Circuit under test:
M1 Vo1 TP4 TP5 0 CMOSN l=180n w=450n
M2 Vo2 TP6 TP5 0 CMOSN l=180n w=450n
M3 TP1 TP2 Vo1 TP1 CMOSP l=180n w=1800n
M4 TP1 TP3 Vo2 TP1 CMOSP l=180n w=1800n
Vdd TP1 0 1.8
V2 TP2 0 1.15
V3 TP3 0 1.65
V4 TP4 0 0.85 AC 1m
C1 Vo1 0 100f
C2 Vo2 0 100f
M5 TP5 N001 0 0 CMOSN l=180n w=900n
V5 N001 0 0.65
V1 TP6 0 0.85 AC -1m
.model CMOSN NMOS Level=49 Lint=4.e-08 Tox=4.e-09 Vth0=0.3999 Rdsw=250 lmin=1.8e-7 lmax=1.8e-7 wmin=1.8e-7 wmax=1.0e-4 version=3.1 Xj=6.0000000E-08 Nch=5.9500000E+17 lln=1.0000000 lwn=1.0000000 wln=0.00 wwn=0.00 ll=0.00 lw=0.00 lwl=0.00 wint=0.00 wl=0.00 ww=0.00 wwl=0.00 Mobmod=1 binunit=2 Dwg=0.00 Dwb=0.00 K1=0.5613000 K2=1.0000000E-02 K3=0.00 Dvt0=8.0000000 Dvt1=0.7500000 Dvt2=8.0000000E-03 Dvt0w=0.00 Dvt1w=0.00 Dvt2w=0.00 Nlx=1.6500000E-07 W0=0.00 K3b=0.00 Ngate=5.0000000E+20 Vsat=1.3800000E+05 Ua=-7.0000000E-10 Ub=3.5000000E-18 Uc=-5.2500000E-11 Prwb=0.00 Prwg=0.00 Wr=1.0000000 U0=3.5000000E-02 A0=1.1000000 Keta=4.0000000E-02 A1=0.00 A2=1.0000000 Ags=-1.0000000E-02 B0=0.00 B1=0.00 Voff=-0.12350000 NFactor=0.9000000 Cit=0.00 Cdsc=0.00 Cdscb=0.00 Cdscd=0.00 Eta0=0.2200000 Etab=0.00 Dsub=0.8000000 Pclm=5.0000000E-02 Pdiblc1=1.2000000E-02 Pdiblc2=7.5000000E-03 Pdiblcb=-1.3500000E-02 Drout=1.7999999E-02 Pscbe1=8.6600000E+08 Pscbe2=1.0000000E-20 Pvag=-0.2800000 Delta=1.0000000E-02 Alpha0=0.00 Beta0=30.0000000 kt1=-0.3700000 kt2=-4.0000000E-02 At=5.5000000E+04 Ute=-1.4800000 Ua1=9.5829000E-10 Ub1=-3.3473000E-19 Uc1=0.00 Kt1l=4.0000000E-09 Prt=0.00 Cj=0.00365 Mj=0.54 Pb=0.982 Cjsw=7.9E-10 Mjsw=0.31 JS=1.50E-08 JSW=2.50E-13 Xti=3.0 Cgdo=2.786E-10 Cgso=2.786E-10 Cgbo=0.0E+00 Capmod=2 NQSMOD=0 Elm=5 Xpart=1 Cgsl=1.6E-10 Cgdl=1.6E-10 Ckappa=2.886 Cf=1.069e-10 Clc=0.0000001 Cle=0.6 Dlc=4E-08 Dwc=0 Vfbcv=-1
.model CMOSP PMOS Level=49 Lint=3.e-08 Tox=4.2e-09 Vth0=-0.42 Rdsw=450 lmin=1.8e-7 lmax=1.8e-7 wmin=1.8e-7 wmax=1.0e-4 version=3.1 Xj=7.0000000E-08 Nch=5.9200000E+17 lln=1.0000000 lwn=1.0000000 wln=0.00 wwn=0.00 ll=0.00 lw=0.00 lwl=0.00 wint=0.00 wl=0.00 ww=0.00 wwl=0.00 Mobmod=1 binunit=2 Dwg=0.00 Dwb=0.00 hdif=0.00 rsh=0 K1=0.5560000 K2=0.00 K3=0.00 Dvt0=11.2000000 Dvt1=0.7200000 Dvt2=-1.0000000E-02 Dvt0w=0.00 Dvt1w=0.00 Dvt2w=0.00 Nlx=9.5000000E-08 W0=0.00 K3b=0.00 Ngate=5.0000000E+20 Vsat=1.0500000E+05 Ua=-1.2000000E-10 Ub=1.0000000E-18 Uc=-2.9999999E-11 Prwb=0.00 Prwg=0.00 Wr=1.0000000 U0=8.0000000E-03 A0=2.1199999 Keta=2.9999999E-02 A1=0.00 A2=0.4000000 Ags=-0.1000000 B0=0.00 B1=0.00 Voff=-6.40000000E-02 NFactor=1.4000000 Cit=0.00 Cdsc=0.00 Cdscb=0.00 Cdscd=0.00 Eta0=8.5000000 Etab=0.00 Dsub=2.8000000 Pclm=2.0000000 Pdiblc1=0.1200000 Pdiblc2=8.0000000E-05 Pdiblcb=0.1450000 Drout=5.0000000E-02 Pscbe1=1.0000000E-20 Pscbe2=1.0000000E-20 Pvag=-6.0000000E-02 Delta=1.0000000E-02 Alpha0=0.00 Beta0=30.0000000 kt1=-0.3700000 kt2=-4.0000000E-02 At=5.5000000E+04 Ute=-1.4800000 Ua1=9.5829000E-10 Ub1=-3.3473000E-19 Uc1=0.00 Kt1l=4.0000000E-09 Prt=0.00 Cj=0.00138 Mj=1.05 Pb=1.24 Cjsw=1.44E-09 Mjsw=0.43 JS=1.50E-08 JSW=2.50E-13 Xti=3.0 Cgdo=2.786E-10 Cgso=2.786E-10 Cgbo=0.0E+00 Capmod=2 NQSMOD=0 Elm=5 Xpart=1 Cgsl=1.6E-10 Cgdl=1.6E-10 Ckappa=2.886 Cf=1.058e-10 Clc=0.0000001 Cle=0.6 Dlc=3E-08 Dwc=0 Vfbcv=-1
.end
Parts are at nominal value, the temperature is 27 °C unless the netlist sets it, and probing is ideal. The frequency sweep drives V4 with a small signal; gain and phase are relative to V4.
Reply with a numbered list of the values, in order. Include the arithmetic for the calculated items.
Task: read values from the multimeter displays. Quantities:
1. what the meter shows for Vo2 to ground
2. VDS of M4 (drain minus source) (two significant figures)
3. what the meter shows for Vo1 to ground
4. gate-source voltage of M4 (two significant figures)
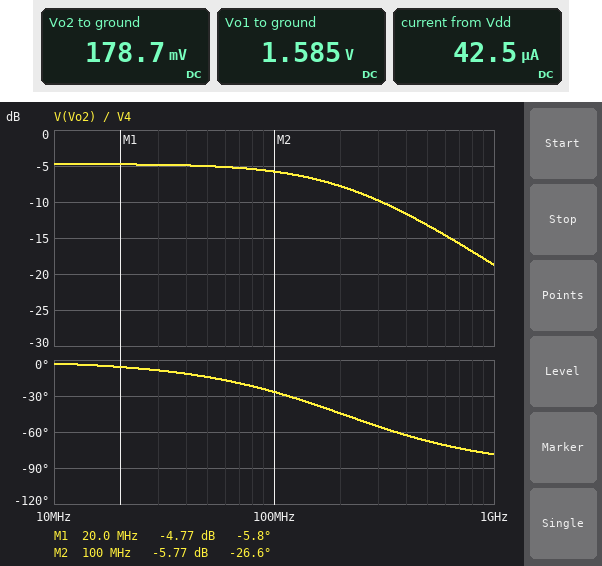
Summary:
1. 178.7 mV
2. 1.8 V - 178.7 mV = 1.6 V
3. 1.585 V
4. 1.65 V - 178.7 mV = 1.5 V
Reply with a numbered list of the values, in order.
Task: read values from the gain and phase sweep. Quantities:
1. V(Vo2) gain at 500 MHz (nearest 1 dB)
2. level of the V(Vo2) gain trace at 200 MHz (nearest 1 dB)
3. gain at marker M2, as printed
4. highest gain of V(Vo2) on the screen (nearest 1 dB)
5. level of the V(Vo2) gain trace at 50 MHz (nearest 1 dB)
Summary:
1. -13 dB
2. -8 dB
3. -5.77 dB
4. -5 dB
5. -5 dB
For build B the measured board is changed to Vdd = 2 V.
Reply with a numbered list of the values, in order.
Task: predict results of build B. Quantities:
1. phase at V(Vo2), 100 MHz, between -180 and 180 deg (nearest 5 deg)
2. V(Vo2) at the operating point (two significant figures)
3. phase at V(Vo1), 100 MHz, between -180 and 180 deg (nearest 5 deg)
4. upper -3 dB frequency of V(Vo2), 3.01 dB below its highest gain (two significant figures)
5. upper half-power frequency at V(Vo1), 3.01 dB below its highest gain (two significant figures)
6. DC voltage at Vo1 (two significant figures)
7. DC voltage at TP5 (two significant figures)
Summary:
1. -40 deg
2. 270 mV
3. -165 deg
4. 110 MHz
5. 710 MHz
6. 1.9 V
7. 220 mV
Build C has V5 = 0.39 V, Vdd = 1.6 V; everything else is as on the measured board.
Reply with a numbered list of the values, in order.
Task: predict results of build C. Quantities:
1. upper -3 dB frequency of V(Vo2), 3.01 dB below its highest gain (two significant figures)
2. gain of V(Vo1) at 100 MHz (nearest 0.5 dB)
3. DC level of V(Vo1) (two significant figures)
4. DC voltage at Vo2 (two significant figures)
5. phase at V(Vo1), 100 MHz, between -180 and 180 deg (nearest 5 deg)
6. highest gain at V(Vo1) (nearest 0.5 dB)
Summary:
1. 14 MHz
2. -23.0 dB
3. 1.6 V
4. 420 mV
5. 155 deg
6. -22.5 dB
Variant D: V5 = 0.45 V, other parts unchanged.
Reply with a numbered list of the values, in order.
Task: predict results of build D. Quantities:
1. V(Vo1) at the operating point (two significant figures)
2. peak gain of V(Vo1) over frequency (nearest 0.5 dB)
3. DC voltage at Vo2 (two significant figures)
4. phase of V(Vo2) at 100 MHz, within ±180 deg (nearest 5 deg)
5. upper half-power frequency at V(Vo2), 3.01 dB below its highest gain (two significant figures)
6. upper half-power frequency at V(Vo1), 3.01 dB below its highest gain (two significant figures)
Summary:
1. 1.8 V
2. -23.0 dB
3. 380 mV
4. -75 deg
5. 31 MHz
6. 480 MHz
